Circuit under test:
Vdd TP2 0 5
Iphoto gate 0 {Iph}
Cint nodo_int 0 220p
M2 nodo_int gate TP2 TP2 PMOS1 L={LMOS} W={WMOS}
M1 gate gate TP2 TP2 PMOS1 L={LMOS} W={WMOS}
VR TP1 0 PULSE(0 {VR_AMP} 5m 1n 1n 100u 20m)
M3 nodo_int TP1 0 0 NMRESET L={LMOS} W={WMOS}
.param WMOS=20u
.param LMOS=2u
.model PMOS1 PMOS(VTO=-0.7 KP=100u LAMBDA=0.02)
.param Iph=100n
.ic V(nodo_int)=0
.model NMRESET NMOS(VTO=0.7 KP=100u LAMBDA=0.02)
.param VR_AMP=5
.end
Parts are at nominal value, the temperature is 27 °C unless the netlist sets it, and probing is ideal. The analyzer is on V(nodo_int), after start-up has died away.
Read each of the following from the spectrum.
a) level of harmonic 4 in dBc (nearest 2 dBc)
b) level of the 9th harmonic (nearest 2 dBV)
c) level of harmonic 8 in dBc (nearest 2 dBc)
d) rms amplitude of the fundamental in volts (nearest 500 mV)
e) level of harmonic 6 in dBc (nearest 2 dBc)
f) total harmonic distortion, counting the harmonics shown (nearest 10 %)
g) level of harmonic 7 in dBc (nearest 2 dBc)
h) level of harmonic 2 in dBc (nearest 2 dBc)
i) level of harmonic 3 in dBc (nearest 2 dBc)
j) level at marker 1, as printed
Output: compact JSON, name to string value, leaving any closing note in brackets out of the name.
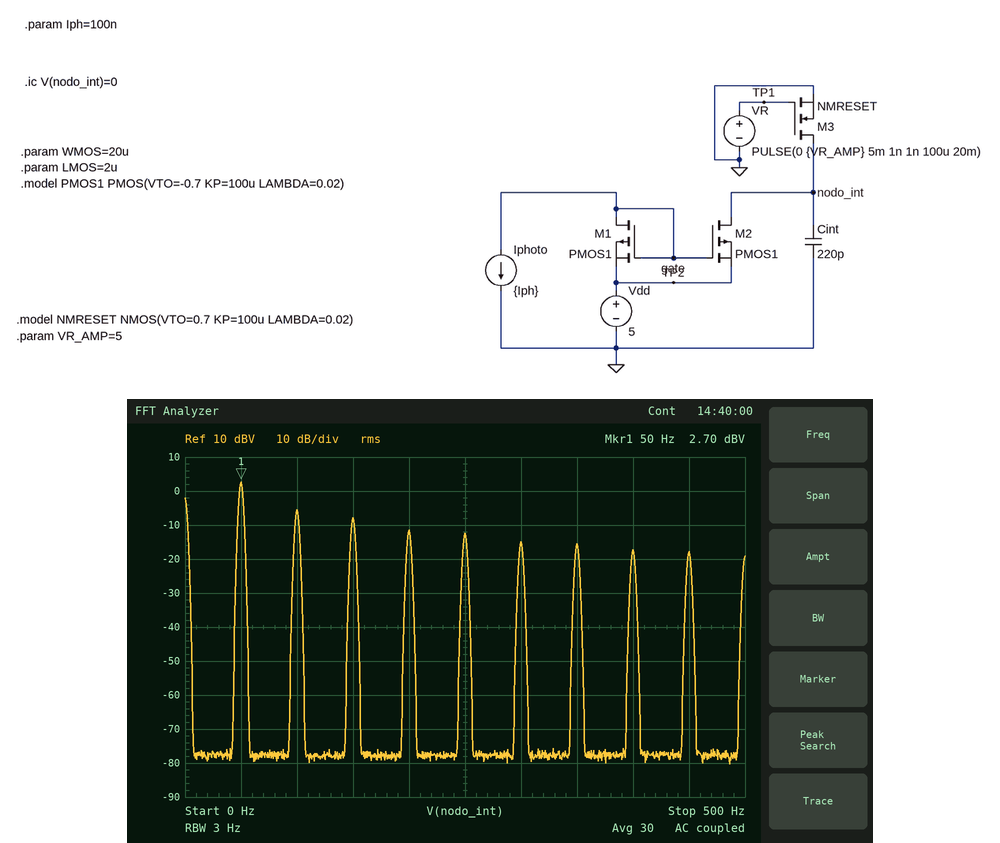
{"level of harmonic 4 in dBc": "-14 dBc", "level of the 9th harmonic": "-18 dBV", "level of harmonic 8 in dBc": "-20 dBc", "rms amplitude of the fundamental in volts": "1.5 V", "level of harmonic 6 in dBc": "-18 dBc", "total harmonic distortion, counting the harmonics shown": "60 %", "level of harmonic 7 in dBc": "-18 dBc", "level of harmonic 2 in dBc": "-8 dBc", "level of harmonic 3 in dBc": "-10 dBc", "level at marker 1, as printed": "2.70 dBV"}
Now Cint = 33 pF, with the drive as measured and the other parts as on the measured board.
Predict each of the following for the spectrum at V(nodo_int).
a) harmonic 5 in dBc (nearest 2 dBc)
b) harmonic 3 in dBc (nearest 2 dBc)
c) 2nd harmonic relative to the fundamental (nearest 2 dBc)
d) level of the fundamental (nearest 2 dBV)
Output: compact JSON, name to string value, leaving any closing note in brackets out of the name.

{"harmonic 5 in dBc": "-2 dBc", "harmonic 3 in dBc": "0 dBc", "2nd harmonic relative to the fundamental": "0 dBc", "level of the fundamental": "-10 dBV"}
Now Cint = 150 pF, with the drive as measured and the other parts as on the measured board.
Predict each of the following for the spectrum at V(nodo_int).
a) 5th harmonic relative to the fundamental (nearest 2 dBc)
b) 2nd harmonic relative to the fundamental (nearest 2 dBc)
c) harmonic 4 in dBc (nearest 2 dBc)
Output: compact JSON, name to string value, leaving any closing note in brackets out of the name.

{"5th harmonic relative to the fundamental": "-14 dBc", "2nd harmonic relative to the fundamental": "-4 dBc", "harmonic 4 in dBc": "-12 dBc"}
